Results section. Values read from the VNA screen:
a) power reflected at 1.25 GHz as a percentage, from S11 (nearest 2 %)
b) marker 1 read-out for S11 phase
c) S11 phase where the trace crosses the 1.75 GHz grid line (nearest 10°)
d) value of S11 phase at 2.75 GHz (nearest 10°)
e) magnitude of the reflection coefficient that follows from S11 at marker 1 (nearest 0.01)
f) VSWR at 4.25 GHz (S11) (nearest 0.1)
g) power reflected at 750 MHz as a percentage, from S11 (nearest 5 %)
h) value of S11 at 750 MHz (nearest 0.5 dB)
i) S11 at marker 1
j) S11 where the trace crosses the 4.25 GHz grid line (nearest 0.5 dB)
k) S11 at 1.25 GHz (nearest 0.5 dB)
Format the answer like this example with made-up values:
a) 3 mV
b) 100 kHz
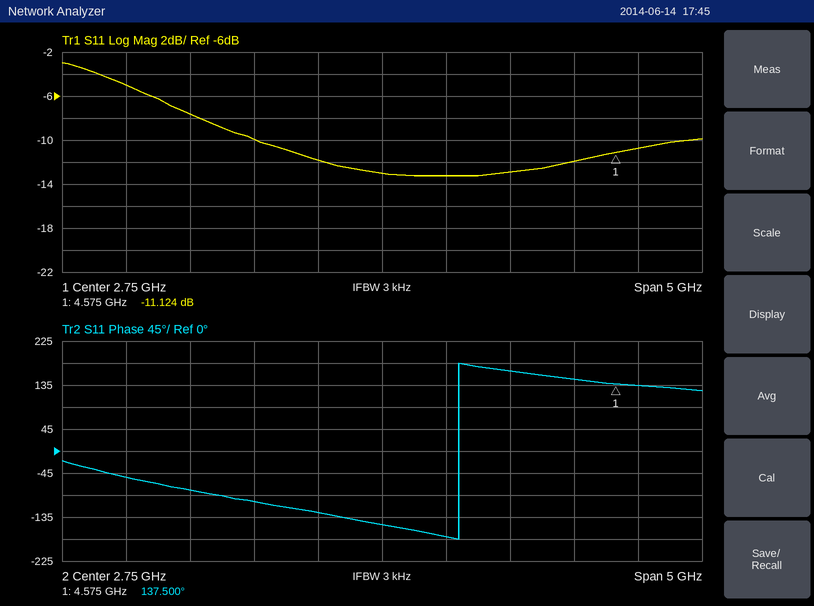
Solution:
a) 18 %
b) 137.500°
c) -100°
d) -150°
e) 0.28
f) 1.7
g) 30 %
h) -5.0 dB
i) -11.124 dB
j) -12.0 dB
k) -7.5 dB
